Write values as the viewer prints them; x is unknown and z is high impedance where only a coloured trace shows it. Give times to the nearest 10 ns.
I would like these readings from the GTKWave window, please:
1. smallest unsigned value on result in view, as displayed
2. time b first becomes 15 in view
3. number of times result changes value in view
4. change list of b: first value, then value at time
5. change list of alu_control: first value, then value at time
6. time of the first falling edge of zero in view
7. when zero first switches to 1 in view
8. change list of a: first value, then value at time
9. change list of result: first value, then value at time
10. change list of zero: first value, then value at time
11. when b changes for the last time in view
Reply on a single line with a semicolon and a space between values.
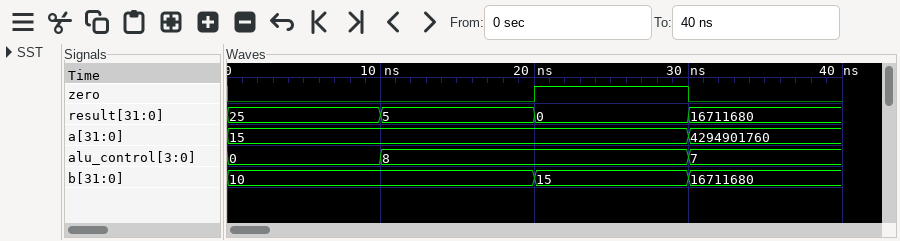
0; 20 ns; 3; 10, 15 at 20 ns, 16711680 at 30 ns; 0, 8 at 10 ns, 7 at 30 ns; 30 ns; 20 ns; 15, 4294901760 at 30 ns; 25, 5 at 10 ns, 0 at 20 ns, 16711680 at 30 ns; 0, 1 at 20 ns, 0 at 30 ns; 30 ns
